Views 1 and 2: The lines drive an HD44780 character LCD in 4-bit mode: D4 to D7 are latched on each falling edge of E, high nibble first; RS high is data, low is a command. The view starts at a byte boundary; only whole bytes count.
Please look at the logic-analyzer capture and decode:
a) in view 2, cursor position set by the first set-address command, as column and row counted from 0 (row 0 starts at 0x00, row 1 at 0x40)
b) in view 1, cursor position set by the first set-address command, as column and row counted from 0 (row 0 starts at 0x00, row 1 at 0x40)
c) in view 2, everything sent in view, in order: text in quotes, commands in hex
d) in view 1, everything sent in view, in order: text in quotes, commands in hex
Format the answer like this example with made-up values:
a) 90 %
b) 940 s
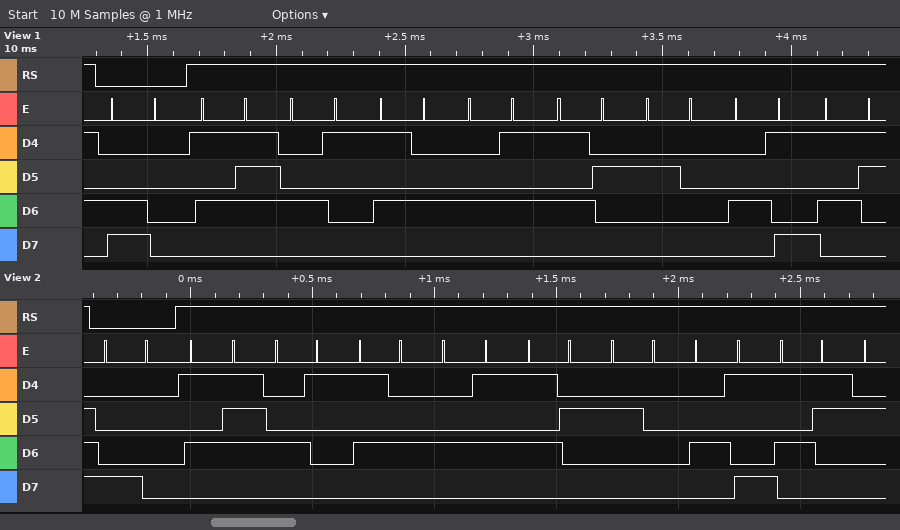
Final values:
a) column 0, row 0
b) column 0, row 1
c) 0x80 "WATER IS"
d) 0xC0 "WATER IS"
